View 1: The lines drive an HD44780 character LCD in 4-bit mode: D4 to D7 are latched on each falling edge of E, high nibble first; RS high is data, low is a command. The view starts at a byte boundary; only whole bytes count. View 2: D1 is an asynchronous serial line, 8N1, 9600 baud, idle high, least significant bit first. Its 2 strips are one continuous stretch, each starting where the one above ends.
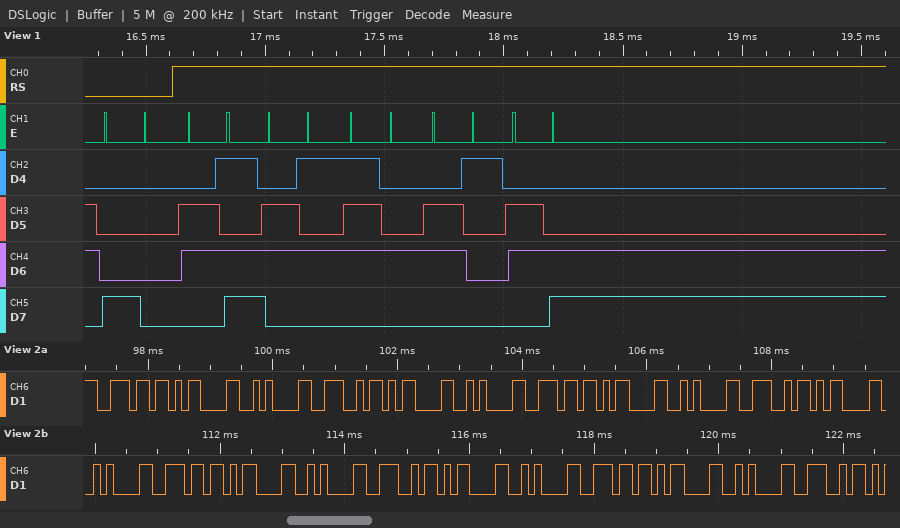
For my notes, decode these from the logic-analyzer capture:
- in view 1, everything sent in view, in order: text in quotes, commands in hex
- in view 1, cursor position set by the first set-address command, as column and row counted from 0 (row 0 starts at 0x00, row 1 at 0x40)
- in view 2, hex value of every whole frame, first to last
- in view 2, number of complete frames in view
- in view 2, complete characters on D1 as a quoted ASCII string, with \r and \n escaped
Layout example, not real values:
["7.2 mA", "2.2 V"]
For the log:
["0x80 \"metal\"", "column 0, row 0", "6E 0D 0A 4E 0D 0A 6E 0D 0A 4E 0D 0A 6E 0D 0A 4E 0D 0A 6E 0D 0A 4E", "22", "\"n\\r\\nN\\r\\nn\\r\\nN\\r\\nn\\r\\nN\\r\\nn\\r\\nN\""]
